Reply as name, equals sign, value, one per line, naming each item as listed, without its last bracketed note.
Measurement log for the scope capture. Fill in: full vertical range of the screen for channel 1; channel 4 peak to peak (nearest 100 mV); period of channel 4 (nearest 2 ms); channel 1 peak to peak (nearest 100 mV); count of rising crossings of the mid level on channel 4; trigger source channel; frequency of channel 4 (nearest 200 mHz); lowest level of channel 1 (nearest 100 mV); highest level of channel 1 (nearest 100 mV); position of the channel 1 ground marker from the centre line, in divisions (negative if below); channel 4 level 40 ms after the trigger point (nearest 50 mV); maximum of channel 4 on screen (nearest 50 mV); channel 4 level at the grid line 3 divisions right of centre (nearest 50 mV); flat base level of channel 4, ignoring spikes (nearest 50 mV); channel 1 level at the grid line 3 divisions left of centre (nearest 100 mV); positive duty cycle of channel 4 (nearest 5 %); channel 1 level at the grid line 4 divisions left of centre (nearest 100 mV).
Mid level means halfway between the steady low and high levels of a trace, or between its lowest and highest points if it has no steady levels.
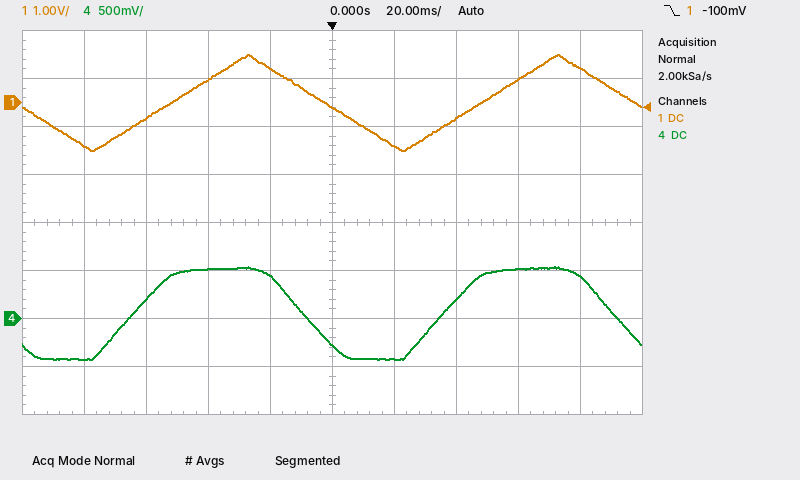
full vertical range of the screen for channel 1 = 8 V
channel 4 peak to peak = 1.00 V
period of channel 4 = 100 ms
channel 1 peak to peak = 2.0 V
count of rising crossings of the mid level on channel 4 = 2
trigger source channel = channel 1
frequency of channel 4 = 10.0 Hz
lowest level of channel 1 = -1.0 V
highest level of channel 1 = 1.0 V
position of the channel 1 ground marker from the centre line, in divisions = +2.5 div
channel 4 level 40 ms after the trigger point = 200 mV
maximum of channel 4 on screen = 550 mV
channel 4 level at the grid line 3 divisions right of centre = 500 mV
flat base level of channel 4, ignoring spikes = -400 mV
channel 1 level at the grid line 3 divisions left of centre = -300 mV
positive duty cycle of channel 4 = 55 %
channel 1 level at the grid line 4 divisions left of centre = -900 mV
